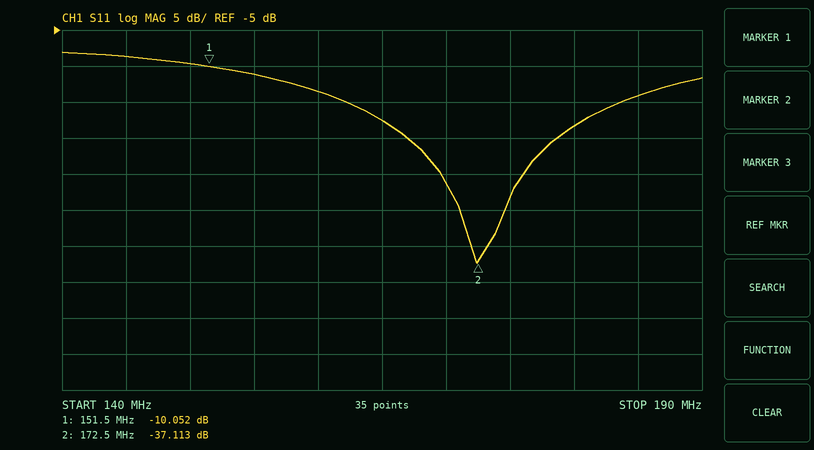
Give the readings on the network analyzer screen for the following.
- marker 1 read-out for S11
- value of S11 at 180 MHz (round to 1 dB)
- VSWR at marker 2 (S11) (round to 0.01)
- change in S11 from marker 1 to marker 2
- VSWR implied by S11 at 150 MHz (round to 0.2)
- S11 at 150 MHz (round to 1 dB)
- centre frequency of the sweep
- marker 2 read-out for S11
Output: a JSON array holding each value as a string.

["-10.052 dB", "-18 dB", "1.03", "-27.061 dB", "2.0", "-10 dB", "165 MHz", "-37.113 dB"]
